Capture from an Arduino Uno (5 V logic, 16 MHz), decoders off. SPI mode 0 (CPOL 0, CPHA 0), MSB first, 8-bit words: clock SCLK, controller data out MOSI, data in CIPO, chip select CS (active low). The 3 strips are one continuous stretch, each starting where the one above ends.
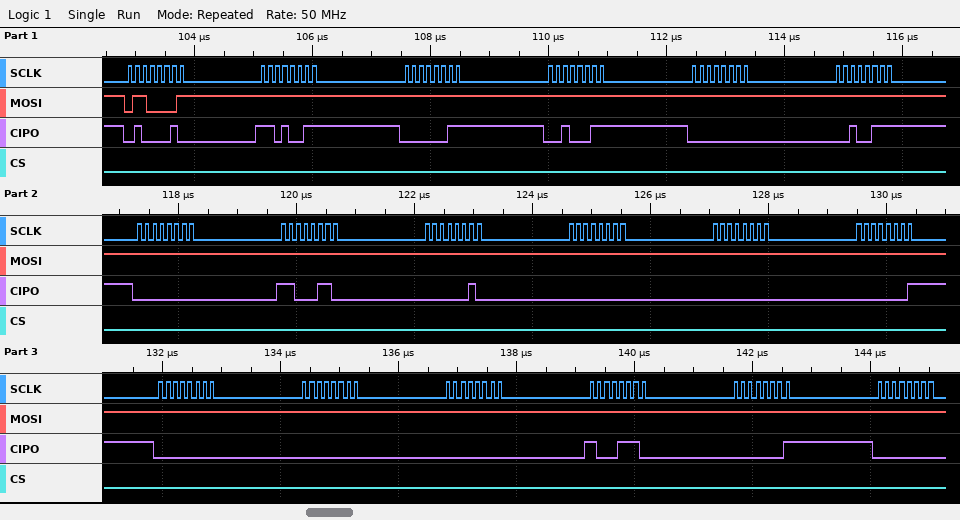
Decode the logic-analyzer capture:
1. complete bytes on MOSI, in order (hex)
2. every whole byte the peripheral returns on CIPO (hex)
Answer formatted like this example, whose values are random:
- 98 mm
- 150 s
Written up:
- 61 FF FF FF FF FF FF FF FF FF FF FF FF FF FF FF FF FF
- 42 D3 03 23 00 27 00 C6 02 00 00 01 00 00 00 8E 01 00
